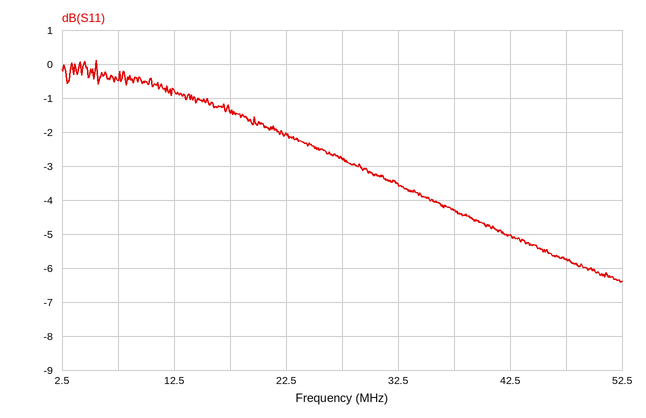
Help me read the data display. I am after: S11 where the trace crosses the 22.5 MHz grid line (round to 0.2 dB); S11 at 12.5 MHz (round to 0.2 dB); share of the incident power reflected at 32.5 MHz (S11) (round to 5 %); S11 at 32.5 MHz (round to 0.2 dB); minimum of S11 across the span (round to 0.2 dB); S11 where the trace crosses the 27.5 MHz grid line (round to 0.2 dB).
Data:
-2.0 dB
-0.8 dB
45 %
-3.6 dB
-6.4 dB
-2.8 dB
